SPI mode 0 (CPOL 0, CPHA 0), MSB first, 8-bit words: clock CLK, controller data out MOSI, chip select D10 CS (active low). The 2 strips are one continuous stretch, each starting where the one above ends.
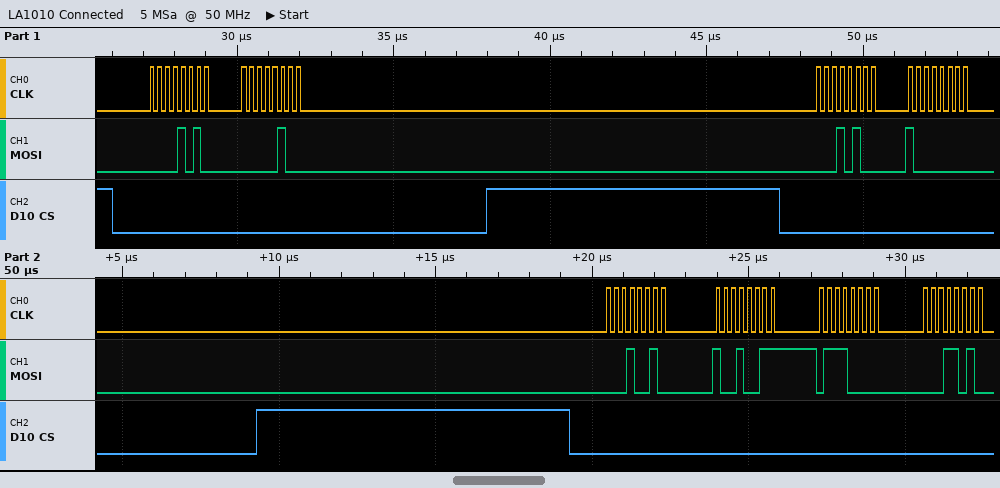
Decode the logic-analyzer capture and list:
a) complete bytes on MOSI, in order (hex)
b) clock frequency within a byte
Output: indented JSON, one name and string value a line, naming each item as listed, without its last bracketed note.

{
  "complete bytes on MOSI, in order": "0A 04 14 80 12 93 70 1A",
  "clock frequency within a byte": "4 MHz"
}
